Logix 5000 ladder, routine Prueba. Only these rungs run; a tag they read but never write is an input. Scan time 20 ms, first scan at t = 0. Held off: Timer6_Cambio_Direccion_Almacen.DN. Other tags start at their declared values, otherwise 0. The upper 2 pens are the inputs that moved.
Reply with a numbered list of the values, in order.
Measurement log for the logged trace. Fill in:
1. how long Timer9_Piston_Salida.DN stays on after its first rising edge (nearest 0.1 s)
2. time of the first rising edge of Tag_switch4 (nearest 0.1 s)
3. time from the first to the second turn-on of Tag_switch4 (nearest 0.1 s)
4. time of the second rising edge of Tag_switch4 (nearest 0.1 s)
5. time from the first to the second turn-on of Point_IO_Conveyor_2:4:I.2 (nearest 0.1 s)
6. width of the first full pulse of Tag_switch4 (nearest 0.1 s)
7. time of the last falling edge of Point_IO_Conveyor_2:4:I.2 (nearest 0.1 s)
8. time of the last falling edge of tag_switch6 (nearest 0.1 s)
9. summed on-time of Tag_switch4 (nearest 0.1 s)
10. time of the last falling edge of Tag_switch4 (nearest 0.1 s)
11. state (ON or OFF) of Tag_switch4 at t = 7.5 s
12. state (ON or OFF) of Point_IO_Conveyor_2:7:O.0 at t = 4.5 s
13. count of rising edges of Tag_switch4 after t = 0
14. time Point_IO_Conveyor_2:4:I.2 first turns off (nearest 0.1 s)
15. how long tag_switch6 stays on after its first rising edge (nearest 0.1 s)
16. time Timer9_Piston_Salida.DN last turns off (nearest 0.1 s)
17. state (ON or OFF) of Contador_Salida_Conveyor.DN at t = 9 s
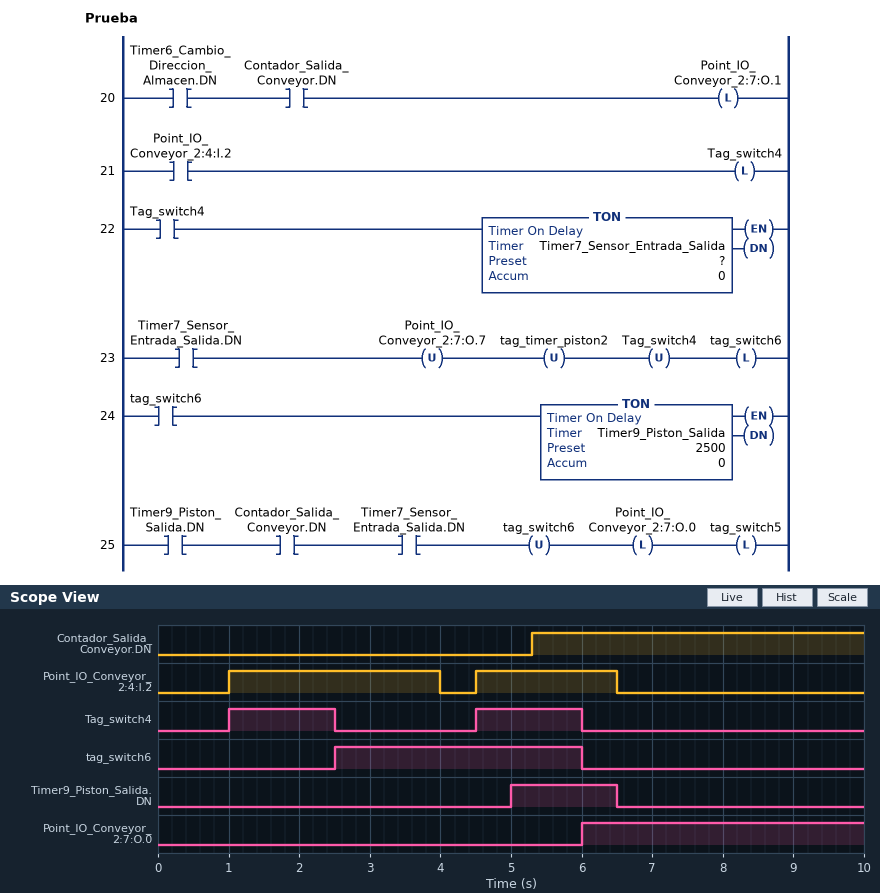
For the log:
1. 1.5 s
2. 1.0 s
3. 3.5 s
4. 4.5 s
5. 3.5 s
6. 1.5 s
7. 6.5 s
8. 6.0 s
9. 3.0 s
10. 6.0 s
11. OFF
12. OFF
13. 2
14. 4.0 s
15. 3.5 s
16. 6.5 s
17. ON
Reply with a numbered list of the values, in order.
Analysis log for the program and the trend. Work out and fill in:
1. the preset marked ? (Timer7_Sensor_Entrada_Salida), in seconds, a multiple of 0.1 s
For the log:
1. 1.5 s
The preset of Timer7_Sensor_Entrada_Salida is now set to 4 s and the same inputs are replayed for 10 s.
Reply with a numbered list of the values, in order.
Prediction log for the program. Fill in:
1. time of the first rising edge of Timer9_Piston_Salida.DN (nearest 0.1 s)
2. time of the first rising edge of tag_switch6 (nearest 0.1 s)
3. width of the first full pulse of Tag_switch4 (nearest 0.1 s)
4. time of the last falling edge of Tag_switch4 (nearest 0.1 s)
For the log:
1. 7.5 s
2. 5.0 s
3. 4.0 s
4. 5.0 s
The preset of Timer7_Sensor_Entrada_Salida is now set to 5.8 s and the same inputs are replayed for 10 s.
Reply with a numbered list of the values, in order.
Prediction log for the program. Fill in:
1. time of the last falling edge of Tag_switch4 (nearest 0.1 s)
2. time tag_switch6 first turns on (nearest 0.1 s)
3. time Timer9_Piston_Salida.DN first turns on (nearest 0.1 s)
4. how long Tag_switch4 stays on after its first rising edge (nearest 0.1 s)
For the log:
1. 6.8 s
2. 6.8 s
3. 9.3 s
4. 5.8 s
